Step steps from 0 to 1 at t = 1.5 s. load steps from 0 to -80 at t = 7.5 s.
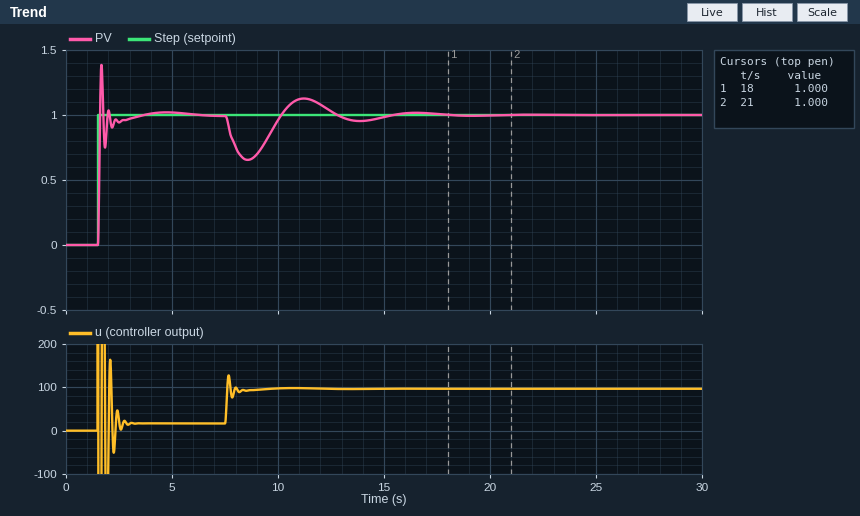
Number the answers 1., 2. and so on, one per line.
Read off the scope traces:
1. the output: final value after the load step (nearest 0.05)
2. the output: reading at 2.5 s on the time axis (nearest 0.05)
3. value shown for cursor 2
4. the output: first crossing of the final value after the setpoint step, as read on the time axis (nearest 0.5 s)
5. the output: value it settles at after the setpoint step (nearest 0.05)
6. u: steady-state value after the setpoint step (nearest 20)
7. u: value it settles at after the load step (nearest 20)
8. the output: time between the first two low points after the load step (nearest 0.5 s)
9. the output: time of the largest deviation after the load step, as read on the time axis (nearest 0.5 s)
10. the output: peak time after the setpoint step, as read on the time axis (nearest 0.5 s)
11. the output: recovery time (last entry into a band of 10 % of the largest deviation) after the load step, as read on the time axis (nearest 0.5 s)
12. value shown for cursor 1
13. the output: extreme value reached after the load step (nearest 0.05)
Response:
1. 1.00
2. 0.95
3. 1.000
4. 1.5 s
5. 1.00
6. 20
7. 100
8. 5.5 s
9. 8.5 s
10. 1.5 s
11. 14.5 s
12. 1.000
13. 0.65
